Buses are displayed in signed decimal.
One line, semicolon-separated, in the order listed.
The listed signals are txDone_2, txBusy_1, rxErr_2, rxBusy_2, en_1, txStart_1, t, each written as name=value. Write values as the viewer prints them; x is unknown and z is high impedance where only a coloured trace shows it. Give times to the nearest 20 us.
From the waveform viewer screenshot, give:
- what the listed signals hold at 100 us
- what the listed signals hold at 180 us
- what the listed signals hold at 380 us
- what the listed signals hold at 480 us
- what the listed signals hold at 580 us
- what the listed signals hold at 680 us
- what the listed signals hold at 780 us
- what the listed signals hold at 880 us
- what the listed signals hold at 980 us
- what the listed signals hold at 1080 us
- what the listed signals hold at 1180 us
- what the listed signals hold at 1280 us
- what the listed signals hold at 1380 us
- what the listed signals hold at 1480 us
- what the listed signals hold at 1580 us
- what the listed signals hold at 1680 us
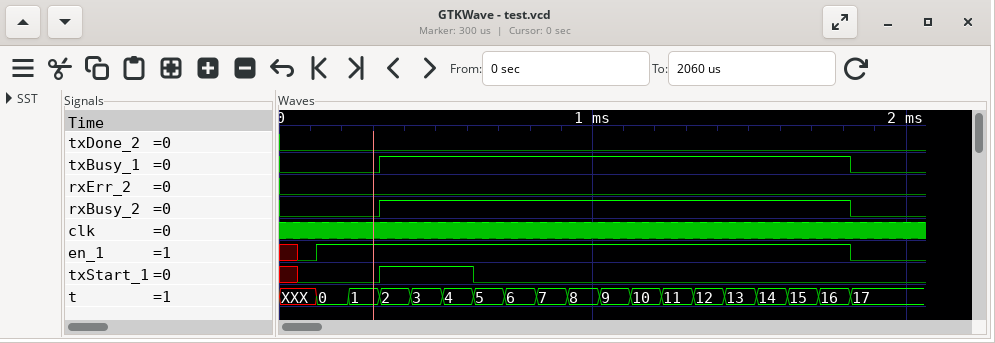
txDone_2=0, txBusy_1=0, rxErr_2=0, rxBusy_2=0, en_1=0, txStart_1=0, t=XXX; txDone_2=0, txBusy_1=0, rxErr_2=0, rxBusy_2=0, en_1=1, txStart_1=0, t=0; txDone_2=0, txBusy_1=1, rxErr_2=0, rxBusy_2=1, en_1=1, txStart_1=1, t=2; txDone_2=0, txBusy_1=1, rxErr_2=0, rxBusy_2=1, en_1=1, txStart_1=1, t=3; txDone_2=0, txBusy_1=1, rxErr_2=0, rxBusy_2=1, en_1=1, txStart_1=1, t=4; txDone_2=0, txBusy_1=1, rxErr_2=0, rxBusy_2=1, en_1=1, txStart_1=0, t=5; txDone_2=0, txBusy_1=1, rxErr_2=0, rxBusy_2=1, en_1=1, txStart_1=0, t=6; txDone_2=0, txBusy_1=1, rxErr_2=0, rxBusy_2=1, en_1=1, txStart_1=0, t=7; txDone_2=0, txBusy_1=1, rxErr_2=0, rxBusy_2=1, en_1=1, txStart_1=0, t=8; txDone_2=0, txBusy_1=1, rxErr_2=0, rxBusy_2=1, en_1=1, txStart_1=0, t=9; txDone_2=0, txBusy_1=1, rxErr_2=0, rxBusy_2=1, en_1=1, txStart_1=0, t=10; txDone_2=0, txBusy_1=1, rxErr_2=0, rxBusy_2=1, en_1=1, txStart_1=0, t=11; txDone_2=0, txBusy_1=1, rxErr_2=0, rxBusy_2=1, en_1=1, txStart_1=0, t=12; txDone_2=0, txBusy_1=1, rxErr_2=0, rxBusy_2=1, en_1=1, txStart_1=0, t=13; txDone_2=0, txBusy_1=1, rxErr_2=0, rxBusy_2=1, en_1=1, txStart_1=0, t=14; txDone_2=0, txBusy_1=1, rxErr_2=0, rxBusy_2=1, en_1=1, txStart_1=0, t=15
